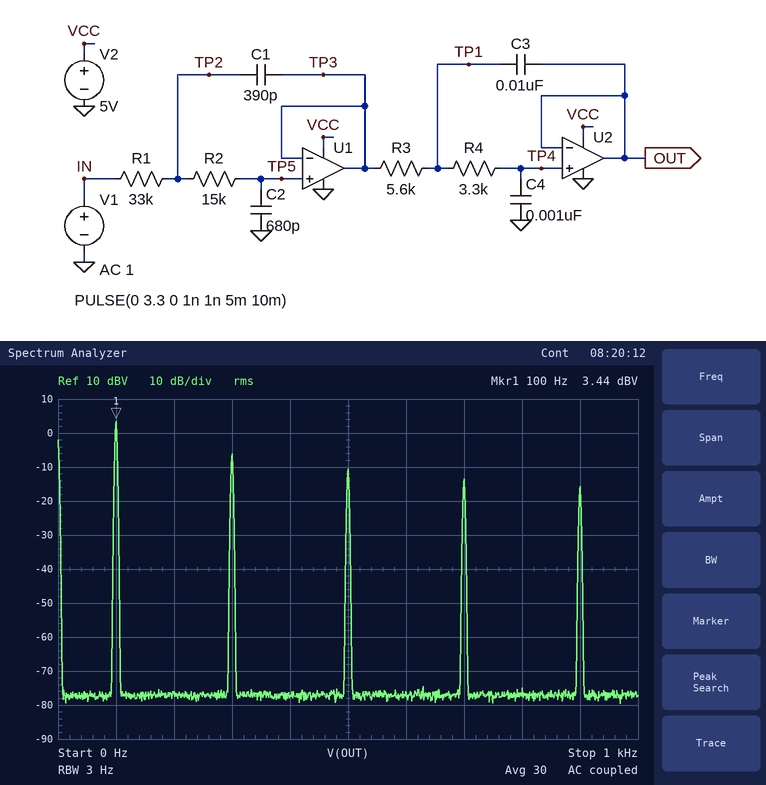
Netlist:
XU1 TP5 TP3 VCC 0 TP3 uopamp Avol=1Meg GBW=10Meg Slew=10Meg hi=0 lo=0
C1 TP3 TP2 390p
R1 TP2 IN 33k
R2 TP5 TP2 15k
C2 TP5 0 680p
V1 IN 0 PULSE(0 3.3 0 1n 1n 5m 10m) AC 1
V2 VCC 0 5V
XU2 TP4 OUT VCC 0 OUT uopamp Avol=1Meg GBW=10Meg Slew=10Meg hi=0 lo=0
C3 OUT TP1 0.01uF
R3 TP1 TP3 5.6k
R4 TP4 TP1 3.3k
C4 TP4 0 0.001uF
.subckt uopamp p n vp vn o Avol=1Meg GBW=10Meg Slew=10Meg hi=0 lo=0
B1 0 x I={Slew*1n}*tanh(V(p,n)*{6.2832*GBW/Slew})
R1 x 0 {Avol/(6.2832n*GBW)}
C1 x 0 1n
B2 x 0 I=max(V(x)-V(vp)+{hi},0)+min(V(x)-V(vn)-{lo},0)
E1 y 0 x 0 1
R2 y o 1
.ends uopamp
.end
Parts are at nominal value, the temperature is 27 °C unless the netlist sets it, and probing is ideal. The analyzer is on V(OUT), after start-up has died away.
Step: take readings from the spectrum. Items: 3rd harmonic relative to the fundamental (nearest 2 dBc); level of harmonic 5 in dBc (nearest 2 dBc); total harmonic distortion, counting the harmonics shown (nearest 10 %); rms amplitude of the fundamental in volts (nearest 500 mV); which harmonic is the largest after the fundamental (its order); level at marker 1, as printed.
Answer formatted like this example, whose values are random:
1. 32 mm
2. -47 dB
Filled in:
1. -10 dBc
2. -14 dBc
3. 40 %
4. 1.5 V
5. 3
6. 3.44 dBV
